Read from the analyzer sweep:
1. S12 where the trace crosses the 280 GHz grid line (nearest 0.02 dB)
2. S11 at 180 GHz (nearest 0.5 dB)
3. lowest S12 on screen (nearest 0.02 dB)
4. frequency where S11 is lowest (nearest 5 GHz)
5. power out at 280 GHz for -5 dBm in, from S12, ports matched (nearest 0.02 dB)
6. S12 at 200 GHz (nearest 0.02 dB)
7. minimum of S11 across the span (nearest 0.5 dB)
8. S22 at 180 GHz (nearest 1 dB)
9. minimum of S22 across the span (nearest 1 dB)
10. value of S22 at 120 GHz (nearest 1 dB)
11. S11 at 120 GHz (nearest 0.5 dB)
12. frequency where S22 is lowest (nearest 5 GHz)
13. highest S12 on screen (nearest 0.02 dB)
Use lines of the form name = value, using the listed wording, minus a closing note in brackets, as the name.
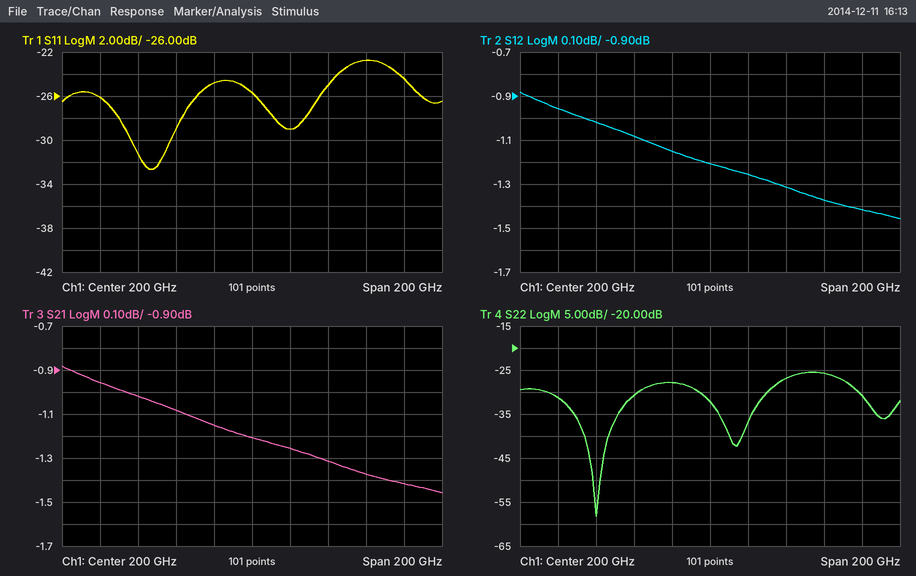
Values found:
S12 where the trace crosses the 280 GHz grid line = -1.42 dB
S11 at 180 GHz = -25.0 dB
lowest S12 on screen = -1.46 dB
frequency where S11 is lowest = 145 GHz
power out at 280 GHz for -5 dBm in, from S12, ports matched = -6.42 dBm
S12 at 200 GHz = -1.20 dB
minimum of S11 across the span = -32.5 dB
S22 at 180 GHz = -28 dB
minimum of S22 across the span = -58 dB
value of S22 at 120 GHz = -31 dB
S11 at 120 GHz = -26.0 dB
frequency where S22 is lowest = 140 GHz
highest S12 on screen = -0.88 dB
